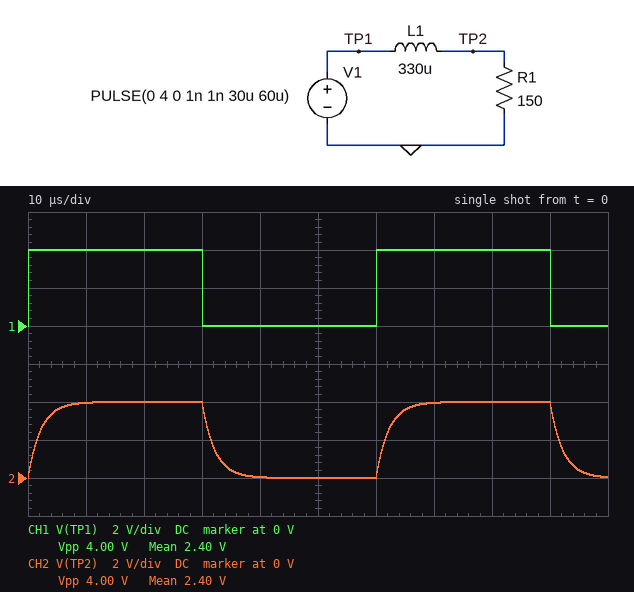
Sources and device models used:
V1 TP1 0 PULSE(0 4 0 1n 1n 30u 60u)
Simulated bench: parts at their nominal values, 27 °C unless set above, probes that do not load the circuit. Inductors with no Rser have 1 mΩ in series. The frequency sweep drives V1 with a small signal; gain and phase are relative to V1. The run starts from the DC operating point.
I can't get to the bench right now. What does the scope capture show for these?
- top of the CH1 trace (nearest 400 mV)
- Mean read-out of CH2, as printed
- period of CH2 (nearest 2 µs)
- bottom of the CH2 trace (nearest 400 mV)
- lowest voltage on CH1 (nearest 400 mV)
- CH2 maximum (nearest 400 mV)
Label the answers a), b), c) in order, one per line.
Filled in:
a) 4.0 V
b) 2.40 V
c) 60 µs
d) 0 V
e) 0 V
f) 4.0 V
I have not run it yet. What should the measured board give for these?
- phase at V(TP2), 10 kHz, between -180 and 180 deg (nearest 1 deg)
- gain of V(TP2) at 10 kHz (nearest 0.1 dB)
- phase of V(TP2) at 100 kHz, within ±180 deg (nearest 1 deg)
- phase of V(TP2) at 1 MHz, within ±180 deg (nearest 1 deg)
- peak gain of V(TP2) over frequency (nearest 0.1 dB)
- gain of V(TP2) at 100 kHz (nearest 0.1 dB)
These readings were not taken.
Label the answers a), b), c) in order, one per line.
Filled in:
a) -8 deg
b) -0.1 dB
c) -54 deg
d) -86 deg
e) 0 dB
f) -4.6 dB
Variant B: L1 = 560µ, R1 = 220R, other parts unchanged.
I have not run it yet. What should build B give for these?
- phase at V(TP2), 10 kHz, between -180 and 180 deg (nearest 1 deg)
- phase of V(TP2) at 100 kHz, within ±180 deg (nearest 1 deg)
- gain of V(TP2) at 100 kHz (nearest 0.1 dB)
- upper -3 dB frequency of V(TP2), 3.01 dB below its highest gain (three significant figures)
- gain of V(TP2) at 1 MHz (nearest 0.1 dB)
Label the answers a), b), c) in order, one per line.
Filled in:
a) -9 deg
b) -58 deg
c) -5.5 dB
d) 62.5 kHz
e) -24.1 dB
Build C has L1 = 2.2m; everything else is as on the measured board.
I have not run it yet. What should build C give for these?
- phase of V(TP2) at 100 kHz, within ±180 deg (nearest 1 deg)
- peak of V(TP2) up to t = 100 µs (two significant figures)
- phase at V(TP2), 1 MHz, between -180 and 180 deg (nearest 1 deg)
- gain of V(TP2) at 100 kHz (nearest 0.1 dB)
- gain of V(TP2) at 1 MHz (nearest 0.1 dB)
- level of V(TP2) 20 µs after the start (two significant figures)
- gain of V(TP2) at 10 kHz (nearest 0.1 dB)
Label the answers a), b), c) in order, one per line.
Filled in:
a) -84 deg
b) 3.5 V
c) -89 deg
d) -19.3 dB
e) -39.3 dB
f) 3.0 V
g) -2.7 dB
